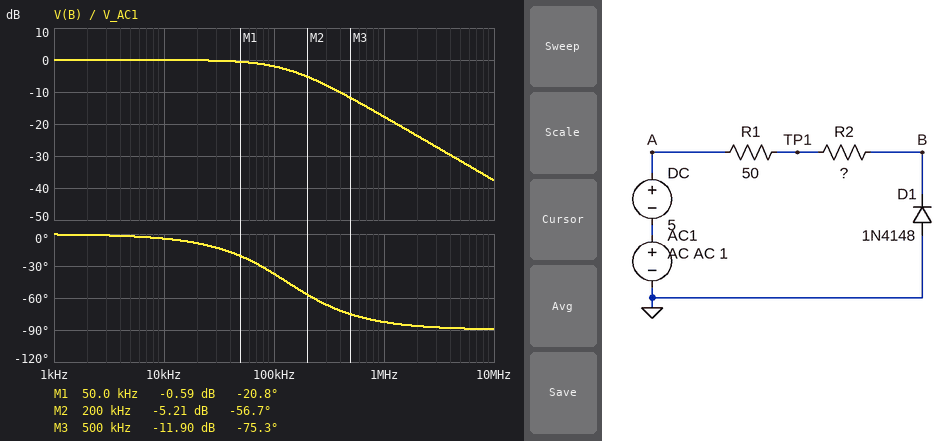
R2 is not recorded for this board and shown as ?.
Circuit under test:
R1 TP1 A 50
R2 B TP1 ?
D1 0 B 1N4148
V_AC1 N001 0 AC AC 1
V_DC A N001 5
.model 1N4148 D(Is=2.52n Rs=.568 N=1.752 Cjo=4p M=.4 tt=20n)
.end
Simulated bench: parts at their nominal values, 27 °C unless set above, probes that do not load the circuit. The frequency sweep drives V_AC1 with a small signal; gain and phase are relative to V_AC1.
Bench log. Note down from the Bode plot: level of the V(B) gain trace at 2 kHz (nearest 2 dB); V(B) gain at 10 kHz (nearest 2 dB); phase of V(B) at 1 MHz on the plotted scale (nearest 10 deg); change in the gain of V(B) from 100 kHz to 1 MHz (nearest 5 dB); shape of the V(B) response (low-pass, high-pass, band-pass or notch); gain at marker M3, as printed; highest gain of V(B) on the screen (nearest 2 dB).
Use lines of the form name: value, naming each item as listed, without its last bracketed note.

level of the V(B) gain trace at 2 kHz: 0 dB
V(B) gain at 10 kHz: 0 dB
phase of V(B) at 1 MHz on the plotted scale: -80 deg
change in the gain of V(B) from 100 kHz to 1 MHz: -15 dB
shape of the V(B) response: low-pass
gain at marker M3, as printed: -11.90 dB
highest gain of V(B) on the screen: 0 dB
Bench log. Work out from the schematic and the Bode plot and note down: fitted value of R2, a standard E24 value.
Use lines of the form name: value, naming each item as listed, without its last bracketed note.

fitted value of R2, a standard E24 value: 620 kΩ
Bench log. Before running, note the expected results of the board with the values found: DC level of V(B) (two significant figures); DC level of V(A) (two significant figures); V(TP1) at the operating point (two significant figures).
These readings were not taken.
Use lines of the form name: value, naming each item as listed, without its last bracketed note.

DC level of V(B): 5.0 V
DC level of V(A): 5.0 V
V(TP1) at the operating point: 5.0 V
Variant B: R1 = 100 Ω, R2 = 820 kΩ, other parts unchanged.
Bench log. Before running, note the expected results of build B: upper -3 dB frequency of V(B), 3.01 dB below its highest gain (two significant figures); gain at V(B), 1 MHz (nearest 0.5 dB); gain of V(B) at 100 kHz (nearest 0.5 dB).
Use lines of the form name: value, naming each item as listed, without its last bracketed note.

upper -3 dB frequency of V(B), 3.01 dB below its highest gain: 99 kHz
gain at V(B), 1 MHz: -20.0 dB
gain of V(B) at 100 kHz: -3.0 dB
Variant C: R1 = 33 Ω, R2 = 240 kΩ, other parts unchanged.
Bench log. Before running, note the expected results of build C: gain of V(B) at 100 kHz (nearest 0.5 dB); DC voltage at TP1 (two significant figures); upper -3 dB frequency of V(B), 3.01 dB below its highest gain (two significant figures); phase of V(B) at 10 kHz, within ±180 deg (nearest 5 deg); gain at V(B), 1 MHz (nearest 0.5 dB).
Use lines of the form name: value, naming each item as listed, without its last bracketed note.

gain of V(B) at 100 kHz: -0.5 dB
DC voltage at TP1: 5.0 V
upper -3 dB frequency of V(B), 3.01 dB below its highest gain: 340 kHz
phase of V(B) at 10 kHz, within ±180 deg: 0 deg
gain at V(B), 1 MHz: -10.0 dB
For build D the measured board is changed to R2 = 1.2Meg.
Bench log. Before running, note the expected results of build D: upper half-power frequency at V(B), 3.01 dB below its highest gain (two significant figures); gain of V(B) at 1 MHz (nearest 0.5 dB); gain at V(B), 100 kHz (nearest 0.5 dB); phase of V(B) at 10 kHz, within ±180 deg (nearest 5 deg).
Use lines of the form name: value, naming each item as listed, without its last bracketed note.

upper half-power frequency at V(B), 3.01 dB below its highest gain: 68 kHz
gain of V(B) at 1 MHz: -23.5 dB
gain at V(B), 100 kHz: -5.0 dB
phase of V(B) at 10 kHz, within ±180 deg: -10 deg
